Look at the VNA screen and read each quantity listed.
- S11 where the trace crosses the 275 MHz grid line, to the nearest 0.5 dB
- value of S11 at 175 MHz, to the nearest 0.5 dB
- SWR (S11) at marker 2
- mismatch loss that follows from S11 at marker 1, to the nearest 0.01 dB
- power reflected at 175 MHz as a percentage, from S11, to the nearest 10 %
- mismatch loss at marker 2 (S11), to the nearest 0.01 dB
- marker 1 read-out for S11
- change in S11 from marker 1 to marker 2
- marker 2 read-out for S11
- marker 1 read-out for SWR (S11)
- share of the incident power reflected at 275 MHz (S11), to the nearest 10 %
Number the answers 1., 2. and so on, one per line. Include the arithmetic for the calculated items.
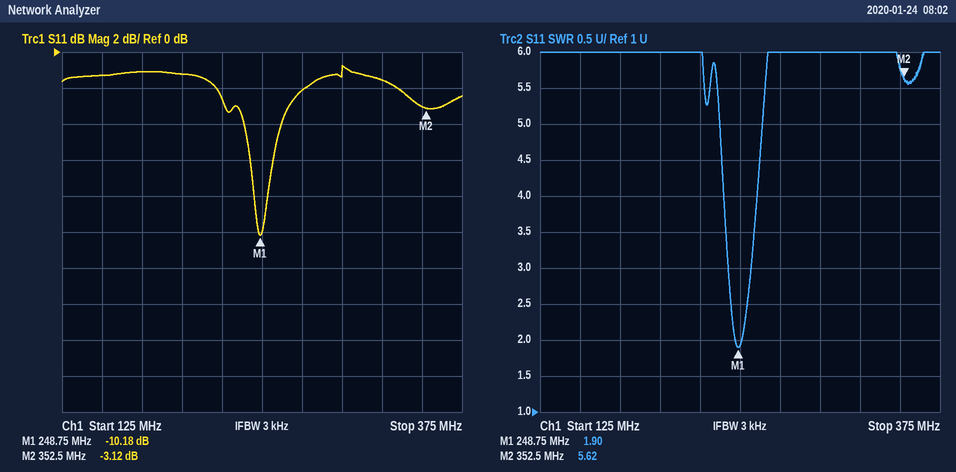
1. -2.0 dB
2. -1.0 dB
3. 5.62
4. −10 log10(1 − 10^(-10.18/10)) ≈ 0.44 dB
5. 10^(-1/10) ≈ 79.4 %, so 80 % to the nearest 10 %
6. −10 log10(1 − 10^(-3.12/10)) ≈ 2.90 dB
7. -10.18 dB
8. -3.12 − (-10.18) = 7.06 dB
9. -3.12 dB
10. 1.90
11. 10^(-2/10) ≈ 63.1 %, so 60 % to the nearest 10 %
